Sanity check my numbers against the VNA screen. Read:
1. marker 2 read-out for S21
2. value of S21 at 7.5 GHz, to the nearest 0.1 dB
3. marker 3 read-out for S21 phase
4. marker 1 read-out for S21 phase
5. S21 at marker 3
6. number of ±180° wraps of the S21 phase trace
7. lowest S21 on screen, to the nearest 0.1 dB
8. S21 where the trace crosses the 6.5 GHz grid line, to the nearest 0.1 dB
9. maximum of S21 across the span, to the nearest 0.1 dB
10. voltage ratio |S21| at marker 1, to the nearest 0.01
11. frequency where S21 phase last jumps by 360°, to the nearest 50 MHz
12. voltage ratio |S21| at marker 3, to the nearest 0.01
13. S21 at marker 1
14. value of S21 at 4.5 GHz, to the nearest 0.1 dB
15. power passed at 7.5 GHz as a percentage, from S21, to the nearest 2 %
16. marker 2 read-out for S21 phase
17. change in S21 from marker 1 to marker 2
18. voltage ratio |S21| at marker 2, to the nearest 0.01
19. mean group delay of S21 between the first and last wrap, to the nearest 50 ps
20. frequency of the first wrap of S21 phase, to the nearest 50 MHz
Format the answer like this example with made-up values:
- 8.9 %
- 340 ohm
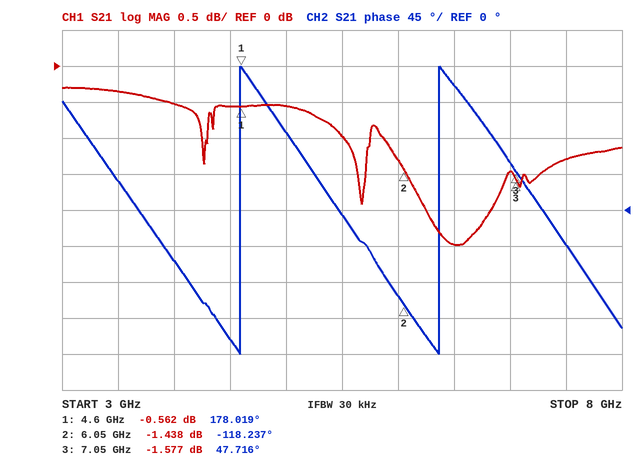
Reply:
- -1.438 dB
- -1.3 dB
- 47.716°
- 178.019°
- -1.577 dB
- 2
- -2.5 dB
- -2.5 dB
- -0.3 dB
- 0.94
- 6.35 GHz
- 0.83
- -0.562 dB
- -0.6 dB
- 74 %
- -118.237°
- -0.876 dB
- 0.85
- 550 ps
- 4.60 GHz
